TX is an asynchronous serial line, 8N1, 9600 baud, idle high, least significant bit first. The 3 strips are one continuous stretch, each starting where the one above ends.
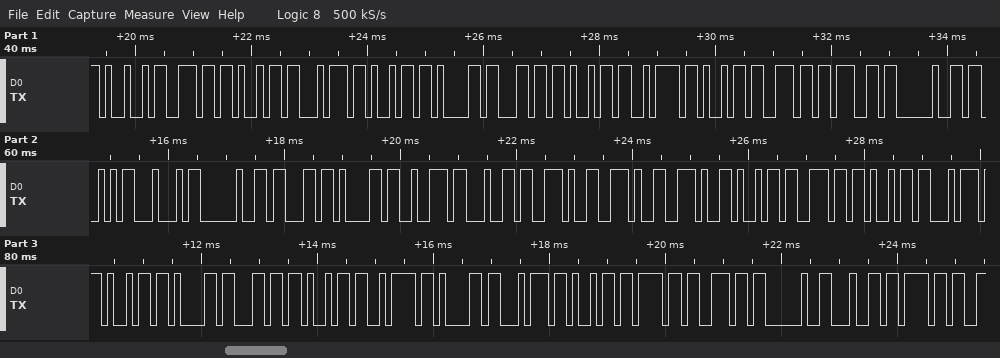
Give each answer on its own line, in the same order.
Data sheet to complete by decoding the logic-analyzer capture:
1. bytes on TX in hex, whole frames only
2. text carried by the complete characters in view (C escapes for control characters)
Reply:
49 6E 69 74 69 61 6C 69 7A 69 6E 67 20 53 44 20 63 61 72 64 2E 2E 2E 69 6E 69 74 69 61 6C 69 7A 61 74 69 6F 6E 20 64 6F
"Initializing SD card...initialization do"
